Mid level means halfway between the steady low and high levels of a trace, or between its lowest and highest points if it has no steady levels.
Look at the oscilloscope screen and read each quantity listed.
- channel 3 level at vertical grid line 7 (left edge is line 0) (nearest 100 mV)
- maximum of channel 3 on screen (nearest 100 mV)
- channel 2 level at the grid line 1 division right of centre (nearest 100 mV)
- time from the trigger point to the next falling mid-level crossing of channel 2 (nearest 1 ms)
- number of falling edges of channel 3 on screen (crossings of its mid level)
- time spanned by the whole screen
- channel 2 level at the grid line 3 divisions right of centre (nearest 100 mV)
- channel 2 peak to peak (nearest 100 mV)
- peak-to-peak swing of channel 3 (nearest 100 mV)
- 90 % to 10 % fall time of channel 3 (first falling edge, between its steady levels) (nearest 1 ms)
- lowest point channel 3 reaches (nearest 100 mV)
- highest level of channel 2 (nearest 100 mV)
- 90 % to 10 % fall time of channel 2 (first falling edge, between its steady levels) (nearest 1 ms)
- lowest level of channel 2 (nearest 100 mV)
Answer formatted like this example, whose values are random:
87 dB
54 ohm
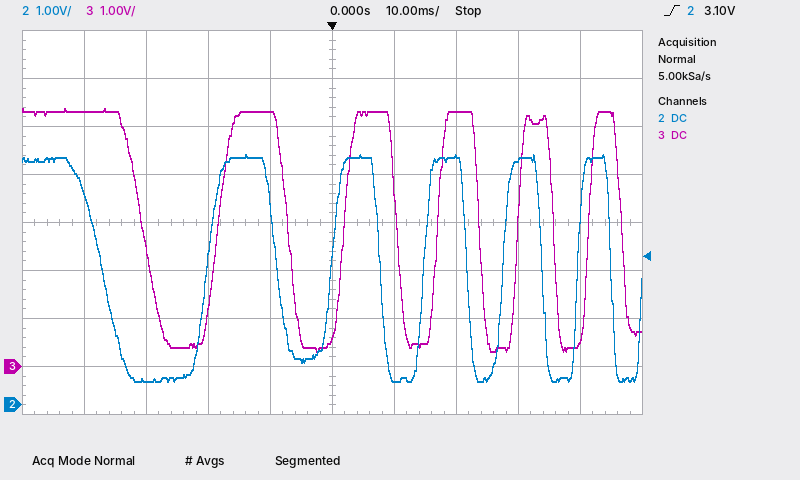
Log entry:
5.3 V
5.4 V
500 mV
8 ms
6
100 ms
5.1 V
4.7 V
5.1 V
6 ms
300 mV
5.2 V
7 ms
500 mV
